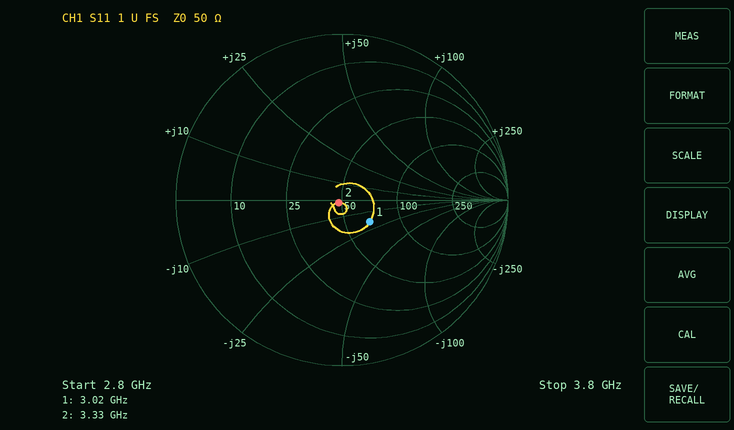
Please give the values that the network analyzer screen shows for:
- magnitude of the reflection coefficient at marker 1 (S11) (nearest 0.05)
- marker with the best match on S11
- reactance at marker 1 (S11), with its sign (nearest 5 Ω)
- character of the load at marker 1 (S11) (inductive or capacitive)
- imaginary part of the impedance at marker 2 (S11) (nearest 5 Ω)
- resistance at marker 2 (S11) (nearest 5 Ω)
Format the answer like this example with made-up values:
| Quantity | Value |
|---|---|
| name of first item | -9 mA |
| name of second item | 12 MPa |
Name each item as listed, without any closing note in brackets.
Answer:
| Quantity | Value |
|---|---|
| magnitude of the reflection coefficient at marker 1 (S11) | 0.20 |
| marker with the best match on S11 | marker 2 |
| reactance at marker 1 (S11), with its sign | -20 Ω |
| character of the load at marker 1 (S11) | capacitive |
| imaginary part of the impedance at marker 2 (S11) | 0 Ω |
| resistance at marker 2 (S11) | 50 Ω |
